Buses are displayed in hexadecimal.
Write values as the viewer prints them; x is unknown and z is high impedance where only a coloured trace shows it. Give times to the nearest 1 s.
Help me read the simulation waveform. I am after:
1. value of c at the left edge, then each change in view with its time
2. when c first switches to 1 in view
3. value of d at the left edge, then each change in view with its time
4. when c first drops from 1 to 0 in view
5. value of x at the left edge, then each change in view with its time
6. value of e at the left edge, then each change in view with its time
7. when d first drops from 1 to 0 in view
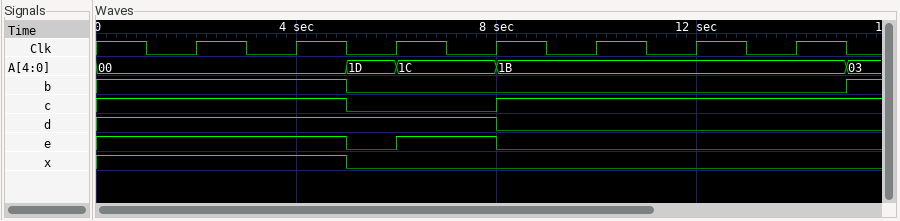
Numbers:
1, 0 at 5 s, 1 at 8 s
8 s
1, 0 at 8 s
5 s
1, 0 at 5 s
1, 0 at 5 s, 1 at 6 s, 0 at 8 s
8 s
